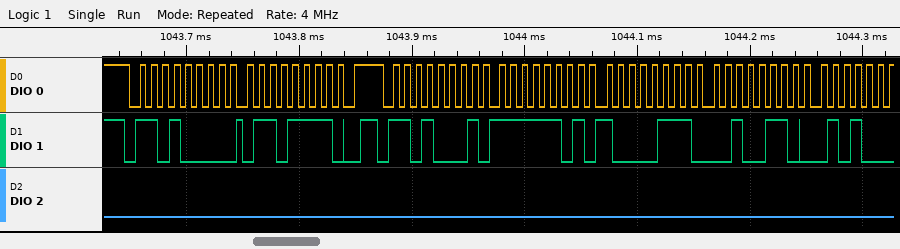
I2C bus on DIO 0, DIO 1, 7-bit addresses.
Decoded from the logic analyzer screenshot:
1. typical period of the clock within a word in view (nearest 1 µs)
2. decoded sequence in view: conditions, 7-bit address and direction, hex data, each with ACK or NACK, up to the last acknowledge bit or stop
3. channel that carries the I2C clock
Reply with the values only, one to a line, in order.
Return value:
10 µs
start, address 68 write ACK, 6F ACK, stop, start, address 68 read ACK, FD ACK, 87 ACK, 26 ACK
DIO 0
